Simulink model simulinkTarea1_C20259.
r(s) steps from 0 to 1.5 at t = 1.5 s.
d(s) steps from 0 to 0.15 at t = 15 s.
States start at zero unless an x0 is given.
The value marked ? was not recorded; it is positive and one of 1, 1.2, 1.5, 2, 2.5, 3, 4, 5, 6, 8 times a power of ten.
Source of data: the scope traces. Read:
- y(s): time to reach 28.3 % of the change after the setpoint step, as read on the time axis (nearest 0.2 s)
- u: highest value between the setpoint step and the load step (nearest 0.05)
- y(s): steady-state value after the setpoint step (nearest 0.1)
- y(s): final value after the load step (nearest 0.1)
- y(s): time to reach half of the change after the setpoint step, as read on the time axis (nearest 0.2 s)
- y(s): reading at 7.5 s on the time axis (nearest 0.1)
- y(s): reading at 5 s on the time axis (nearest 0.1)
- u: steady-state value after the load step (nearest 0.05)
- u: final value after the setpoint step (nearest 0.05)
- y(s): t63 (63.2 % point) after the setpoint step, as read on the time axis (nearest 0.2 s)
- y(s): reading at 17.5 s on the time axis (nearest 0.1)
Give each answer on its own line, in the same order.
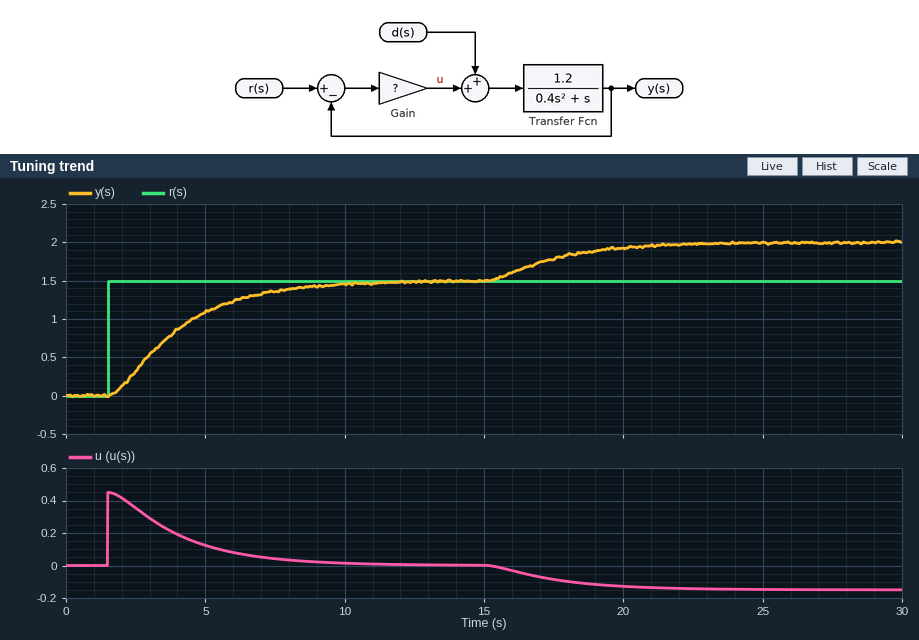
2.8 s
0.45
1.5
2.0
3.6 s
1.4
1.1
-0.15
0.00
4.4 s
1.8
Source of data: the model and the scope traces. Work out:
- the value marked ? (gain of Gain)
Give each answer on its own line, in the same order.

0.3
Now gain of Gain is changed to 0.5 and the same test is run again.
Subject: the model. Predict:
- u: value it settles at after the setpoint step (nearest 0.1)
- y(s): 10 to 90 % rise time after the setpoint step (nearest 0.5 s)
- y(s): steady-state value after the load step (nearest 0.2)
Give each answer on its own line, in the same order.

0.0
3.0 s
1.8
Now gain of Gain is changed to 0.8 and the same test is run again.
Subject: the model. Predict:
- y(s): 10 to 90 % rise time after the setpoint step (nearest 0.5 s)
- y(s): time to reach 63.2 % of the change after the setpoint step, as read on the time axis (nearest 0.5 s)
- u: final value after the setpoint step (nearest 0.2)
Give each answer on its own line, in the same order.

1.5 s
2.5 s
0.0
